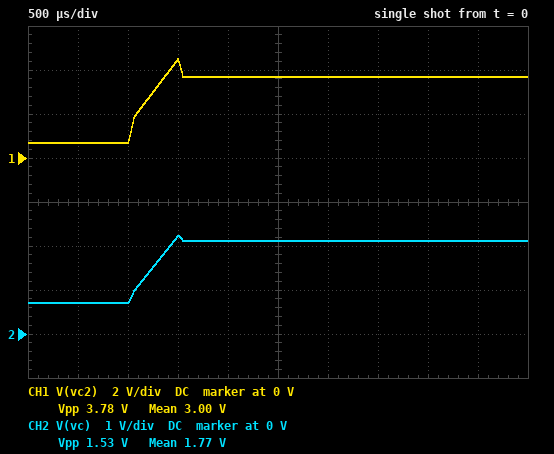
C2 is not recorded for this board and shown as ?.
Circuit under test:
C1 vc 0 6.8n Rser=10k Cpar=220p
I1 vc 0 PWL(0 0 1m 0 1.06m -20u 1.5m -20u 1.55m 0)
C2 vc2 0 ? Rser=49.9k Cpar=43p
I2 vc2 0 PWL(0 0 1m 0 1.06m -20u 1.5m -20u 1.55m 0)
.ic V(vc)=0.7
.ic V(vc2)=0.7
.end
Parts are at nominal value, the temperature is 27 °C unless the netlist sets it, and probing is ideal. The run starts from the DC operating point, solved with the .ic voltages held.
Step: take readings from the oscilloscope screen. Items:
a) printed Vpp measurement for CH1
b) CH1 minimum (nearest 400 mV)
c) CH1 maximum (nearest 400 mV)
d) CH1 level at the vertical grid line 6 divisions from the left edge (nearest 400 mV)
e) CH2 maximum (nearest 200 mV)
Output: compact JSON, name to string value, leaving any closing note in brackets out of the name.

{"printed Vpp measurement for CH1": "3.78 V", "CH1 minimum": "800 mV", "CH1 maximum": "4.4 V", "CH1 level at the vertical grid line 6 divisions from the left edge": "3.6 V", "CH2 maximum": "2.2 V"}
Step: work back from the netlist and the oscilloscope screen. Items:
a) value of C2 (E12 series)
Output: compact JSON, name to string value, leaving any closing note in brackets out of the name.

{"value of C2": "3.3 nF"}
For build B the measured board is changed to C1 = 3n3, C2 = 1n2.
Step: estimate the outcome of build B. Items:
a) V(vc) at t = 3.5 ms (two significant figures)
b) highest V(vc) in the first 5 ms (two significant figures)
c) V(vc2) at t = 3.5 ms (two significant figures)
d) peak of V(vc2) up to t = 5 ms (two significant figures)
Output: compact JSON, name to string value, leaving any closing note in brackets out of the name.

{"V(vc) at t = 3.5 ms": "3.5 V", "highest V(vc) in the first 5 ms": "3.6 V", "V(vc2) at t = 3.5 ms": "8.7 V", "peak of V(vc2) up to t = 5 ms": "9.2 V"}
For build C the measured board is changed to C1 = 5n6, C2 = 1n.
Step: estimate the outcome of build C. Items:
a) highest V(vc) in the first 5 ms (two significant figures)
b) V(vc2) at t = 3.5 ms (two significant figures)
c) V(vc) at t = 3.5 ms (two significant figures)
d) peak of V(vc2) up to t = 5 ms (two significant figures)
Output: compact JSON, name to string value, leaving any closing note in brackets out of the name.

{"highest V(vc) in the first 5 ms": "2.5 V", "V(vc2) at t = 3.5 ms": "10 V", "V(vc) at t = 3.5 ms": "2.4 V", "peak of V(vc2) up to t = 5 ms": "11 V"}
